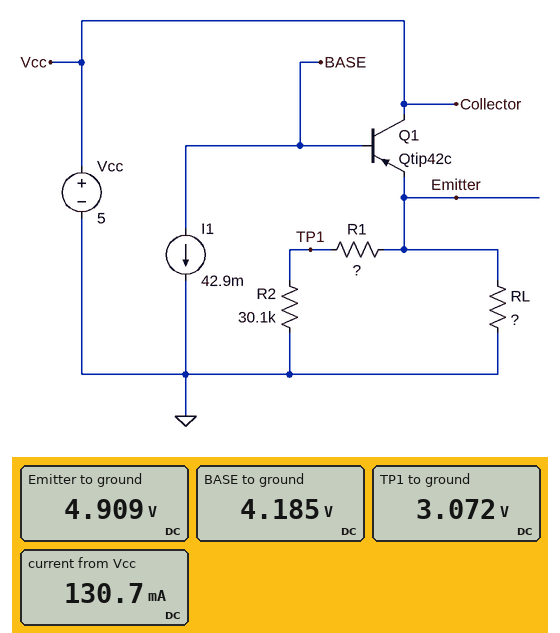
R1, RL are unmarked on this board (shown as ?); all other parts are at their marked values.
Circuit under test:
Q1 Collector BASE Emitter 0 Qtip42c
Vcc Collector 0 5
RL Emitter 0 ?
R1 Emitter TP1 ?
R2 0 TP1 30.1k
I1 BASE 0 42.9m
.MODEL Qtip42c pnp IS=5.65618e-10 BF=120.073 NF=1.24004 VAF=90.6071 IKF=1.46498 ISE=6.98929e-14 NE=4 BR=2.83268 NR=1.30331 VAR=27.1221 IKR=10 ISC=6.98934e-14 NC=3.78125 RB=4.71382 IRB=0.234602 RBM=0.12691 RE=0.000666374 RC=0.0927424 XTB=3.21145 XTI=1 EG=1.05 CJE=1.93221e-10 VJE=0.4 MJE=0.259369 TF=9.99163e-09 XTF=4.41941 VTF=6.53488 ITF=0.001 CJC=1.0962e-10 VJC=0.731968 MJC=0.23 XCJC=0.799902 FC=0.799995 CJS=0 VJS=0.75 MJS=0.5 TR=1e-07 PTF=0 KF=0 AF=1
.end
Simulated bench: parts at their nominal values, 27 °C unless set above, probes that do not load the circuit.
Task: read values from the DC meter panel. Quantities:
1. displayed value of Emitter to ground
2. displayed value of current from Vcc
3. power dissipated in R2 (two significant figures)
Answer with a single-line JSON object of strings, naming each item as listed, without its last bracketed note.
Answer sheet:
{"displayed value of Emitter to ground": "4.909 V", "displayed value of current from Vcc": "130.7 mA", "power dissipated in R2": "310 µW"}
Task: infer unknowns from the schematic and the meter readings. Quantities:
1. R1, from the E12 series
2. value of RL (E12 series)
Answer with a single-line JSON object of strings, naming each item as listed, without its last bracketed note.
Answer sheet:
{"R1, from the E12 series": "18 kΩ", "value of RL": "56 Ω"}
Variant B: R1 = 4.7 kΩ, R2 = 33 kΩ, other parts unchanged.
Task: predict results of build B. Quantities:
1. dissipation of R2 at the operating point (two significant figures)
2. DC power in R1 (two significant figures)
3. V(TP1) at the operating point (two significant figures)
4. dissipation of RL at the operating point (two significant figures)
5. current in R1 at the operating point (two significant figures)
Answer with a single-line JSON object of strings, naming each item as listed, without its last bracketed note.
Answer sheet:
{"dissipation of R2 at the operating point": "560 µW", "DC power in R1": "80 µW", "V(TP1) at the operating point": "4.3 V", "dissipation of RL at the operating point": "430 mW", "current in R1 at the operating point": "130 µA"}
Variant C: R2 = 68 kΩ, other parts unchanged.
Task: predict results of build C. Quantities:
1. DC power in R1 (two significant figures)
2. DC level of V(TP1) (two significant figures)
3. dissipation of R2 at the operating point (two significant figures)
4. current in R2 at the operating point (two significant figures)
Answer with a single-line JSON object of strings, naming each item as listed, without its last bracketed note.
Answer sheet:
{"DC power in R1": "59 µW", "DC level of V(TP1)": "3.9 V", "dissipation of R2 at the operating point": "220 µW", "current in R2 at the operating point": "57 µA"}
